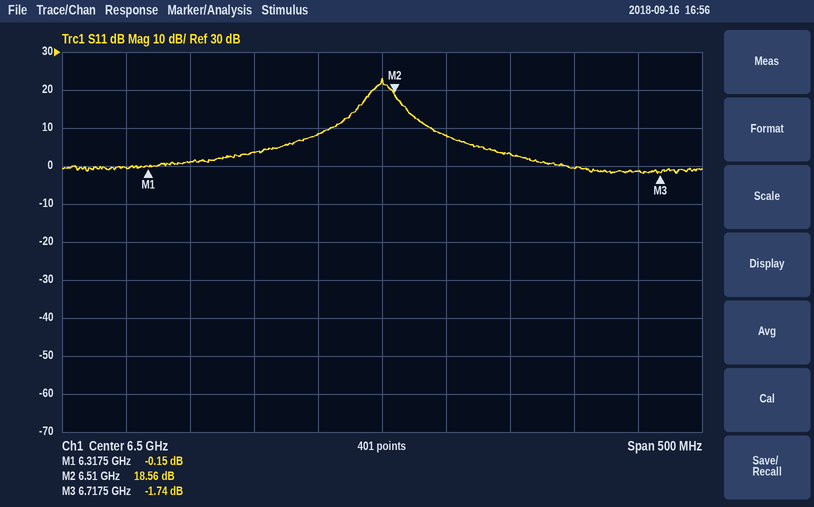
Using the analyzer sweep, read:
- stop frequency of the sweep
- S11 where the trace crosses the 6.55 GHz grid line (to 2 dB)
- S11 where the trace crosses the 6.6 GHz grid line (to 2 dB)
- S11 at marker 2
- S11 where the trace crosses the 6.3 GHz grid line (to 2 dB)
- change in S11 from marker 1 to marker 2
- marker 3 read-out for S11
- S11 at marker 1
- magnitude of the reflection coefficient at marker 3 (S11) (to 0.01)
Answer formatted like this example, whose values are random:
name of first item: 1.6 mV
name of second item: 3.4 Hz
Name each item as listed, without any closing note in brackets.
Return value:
stop frequency of the sweep: 6.75 GHz
S11 where the trace crosses the 6.55 GHz grid line: 8 dB
S11 where the trace crosses the 6.6 GHz grid line: 4 dB
S11 at marker 2: 18.56 dB
S11 where the trace crosses the 6.3 GHz grid line: 0 dB
change in S11 from marker 1 to marker 2: 18.71 dB
marker 3 read-out for S11: -1.74 dB
S11 at marker 1: -0.15 dB
magnitude of the reflection coefficient at marker 3 (S11): 0.82
